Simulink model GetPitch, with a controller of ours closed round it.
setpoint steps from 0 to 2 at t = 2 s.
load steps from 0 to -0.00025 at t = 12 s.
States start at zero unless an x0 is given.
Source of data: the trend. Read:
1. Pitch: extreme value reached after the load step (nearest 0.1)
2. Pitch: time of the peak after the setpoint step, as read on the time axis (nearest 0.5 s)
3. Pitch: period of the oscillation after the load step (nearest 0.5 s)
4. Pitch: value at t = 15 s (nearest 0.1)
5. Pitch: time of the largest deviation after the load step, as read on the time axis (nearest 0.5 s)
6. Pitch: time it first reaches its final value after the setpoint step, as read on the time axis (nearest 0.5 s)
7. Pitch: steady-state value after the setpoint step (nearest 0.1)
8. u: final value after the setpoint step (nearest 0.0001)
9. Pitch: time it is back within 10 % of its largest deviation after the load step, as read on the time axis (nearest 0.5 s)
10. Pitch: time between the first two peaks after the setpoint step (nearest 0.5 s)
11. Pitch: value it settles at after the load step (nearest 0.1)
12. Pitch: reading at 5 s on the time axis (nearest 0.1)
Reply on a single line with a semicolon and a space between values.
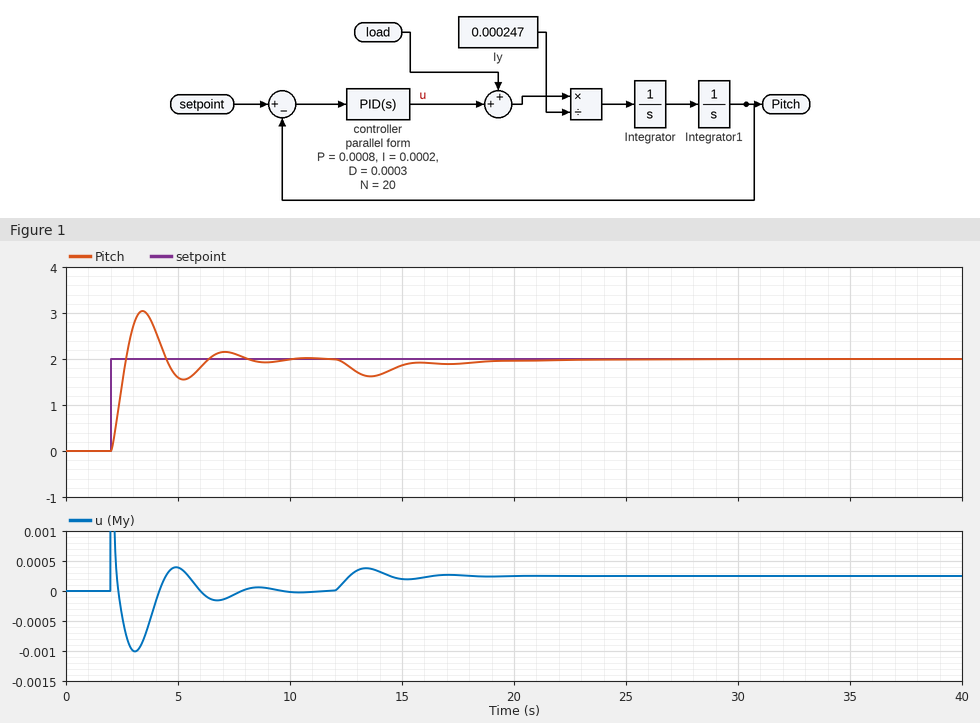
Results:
1.6; 3.5 s; 3.5 s; 1.9; 13.5 s; 2.5 s; 2.0; 0.0000; 20.5 s; 3.5 s; 2.0; 1.6
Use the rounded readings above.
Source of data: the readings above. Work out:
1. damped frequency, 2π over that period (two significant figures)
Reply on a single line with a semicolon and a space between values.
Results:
1.8 rad/s
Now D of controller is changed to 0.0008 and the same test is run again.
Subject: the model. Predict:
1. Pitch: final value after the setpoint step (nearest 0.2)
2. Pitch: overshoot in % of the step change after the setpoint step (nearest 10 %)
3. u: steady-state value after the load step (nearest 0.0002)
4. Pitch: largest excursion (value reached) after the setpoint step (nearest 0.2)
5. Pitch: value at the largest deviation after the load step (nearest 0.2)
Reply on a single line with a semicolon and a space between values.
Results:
2.0; 20 %; 0.0002; 2.4; 1.8
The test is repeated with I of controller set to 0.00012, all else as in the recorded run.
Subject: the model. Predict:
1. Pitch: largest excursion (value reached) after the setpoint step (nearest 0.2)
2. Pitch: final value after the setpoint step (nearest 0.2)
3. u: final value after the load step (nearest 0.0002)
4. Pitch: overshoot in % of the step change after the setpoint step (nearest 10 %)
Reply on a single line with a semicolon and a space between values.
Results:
3.0; 2.0; 0.0002; 50 %
